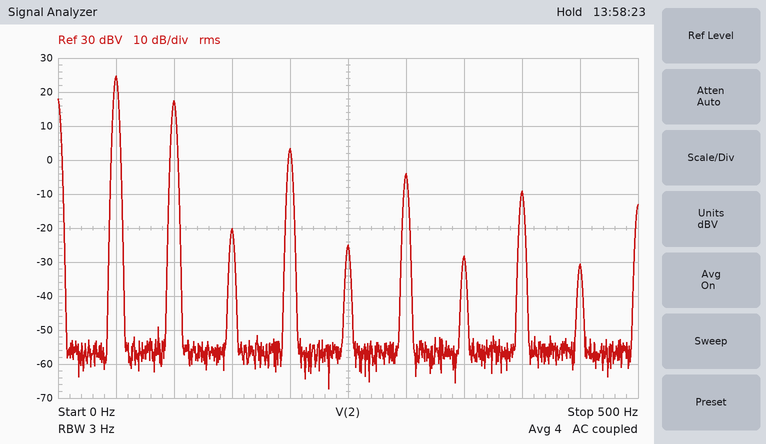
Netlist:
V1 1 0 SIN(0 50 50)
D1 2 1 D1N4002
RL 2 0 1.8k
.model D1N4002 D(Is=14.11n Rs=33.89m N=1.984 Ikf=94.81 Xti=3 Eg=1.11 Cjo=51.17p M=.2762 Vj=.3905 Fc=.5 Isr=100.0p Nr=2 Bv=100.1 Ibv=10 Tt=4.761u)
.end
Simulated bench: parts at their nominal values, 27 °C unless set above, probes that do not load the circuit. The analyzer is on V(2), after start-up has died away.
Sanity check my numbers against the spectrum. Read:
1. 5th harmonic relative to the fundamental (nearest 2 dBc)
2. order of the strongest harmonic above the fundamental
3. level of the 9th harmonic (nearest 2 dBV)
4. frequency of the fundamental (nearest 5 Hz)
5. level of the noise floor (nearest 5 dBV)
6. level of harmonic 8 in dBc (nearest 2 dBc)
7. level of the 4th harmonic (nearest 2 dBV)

-50 dBc
2
-30 dBV
50 Hz
-55 dBV
-34 dBc
4 dBV
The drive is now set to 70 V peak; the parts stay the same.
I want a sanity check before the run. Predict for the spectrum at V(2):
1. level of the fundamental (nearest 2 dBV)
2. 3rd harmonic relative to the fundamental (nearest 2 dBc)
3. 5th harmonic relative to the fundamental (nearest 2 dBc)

28 dBV
-48 dBc
-52 dBc
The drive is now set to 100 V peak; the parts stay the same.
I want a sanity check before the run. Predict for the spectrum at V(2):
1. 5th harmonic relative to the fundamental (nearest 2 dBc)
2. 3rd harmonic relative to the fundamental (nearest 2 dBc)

-58 dBc
-50 dBc
